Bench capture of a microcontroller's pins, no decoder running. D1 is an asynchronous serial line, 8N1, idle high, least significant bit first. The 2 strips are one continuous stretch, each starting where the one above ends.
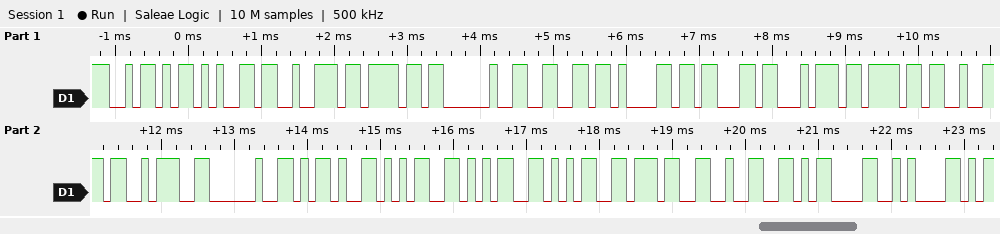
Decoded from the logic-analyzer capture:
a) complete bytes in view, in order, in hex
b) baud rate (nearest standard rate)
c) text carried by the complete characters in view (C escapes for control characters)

0x5A 0x65 0x72 0x6F 0x20 0x66 0x61 0x63 0x74 0x6F 0x72 0x3A 0x20 0x2D 0x35 0x35 0x35 0x37 0x32 0x0D 0x0A
9600 baud
"Zero factor: -55572\r\n"
